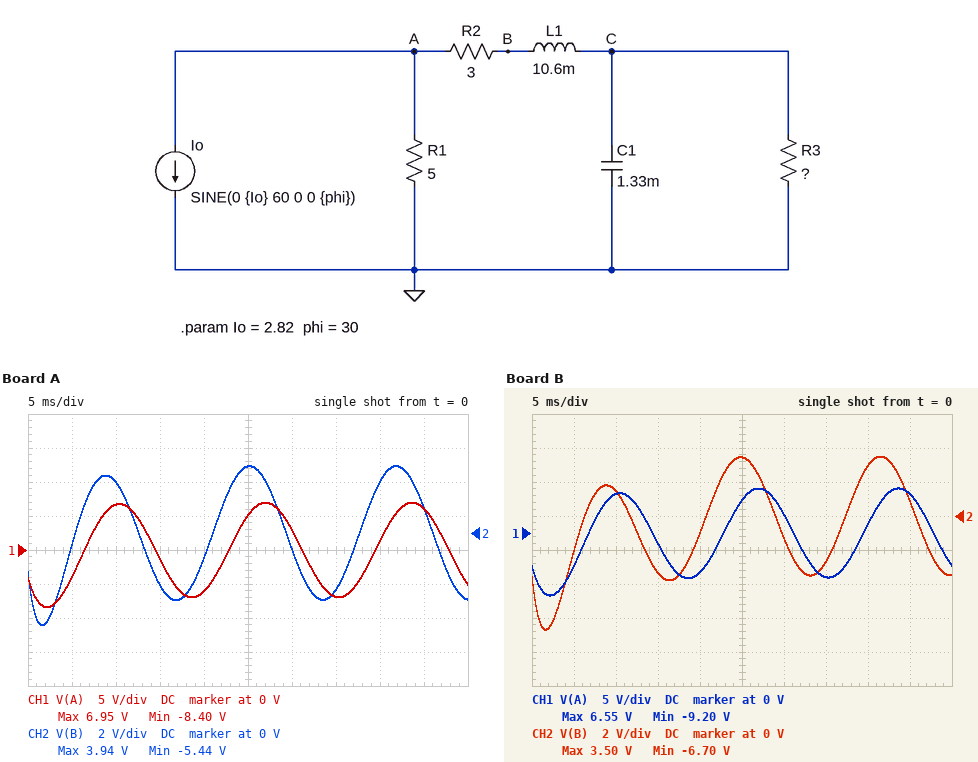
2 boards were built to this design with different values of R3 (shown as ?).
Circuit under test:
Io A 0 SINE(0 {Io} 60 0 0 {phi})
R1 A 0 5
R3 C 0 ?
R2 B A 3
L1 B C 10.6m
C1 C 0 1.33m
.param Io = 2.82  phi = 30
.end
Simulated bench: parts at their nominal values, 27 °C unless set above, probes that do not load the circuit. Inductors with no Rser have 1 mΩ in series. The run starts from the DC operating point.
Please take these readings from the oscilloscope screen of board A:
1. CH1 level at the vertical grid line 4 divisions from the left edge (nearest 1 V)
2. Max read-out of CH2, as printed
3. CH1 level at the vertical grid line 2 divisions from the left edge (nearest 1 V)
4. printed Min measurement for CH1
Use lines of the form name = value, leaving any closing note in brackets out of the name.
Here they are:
CH1 level at the vertical grid line 4 divisions from the left edge = -6 V
Max read-out of CH2, as printed = 3.94 V
CH1 level at the vertical grid line 2 divisions from the left edge = 7 V
printed Min measurement for CH1 = -8.40 V
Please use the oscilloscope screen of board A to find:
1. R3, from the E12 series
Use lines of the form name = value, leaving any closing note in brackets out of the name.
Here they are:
R3, from the E12 series = 3.9 Ω
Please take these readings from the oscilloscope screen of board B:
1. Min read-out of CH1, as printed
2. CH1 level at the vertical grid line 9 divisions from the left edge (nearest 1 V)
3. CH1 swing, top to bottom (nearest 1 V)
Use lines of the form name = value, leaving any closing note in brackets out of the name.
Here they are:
Min read-out of CH1, as printed = -9.20 V
CH1 level at the vertical grid line 9 divisions from the left edge = 6 V
CH1 swing, top to bottom = 16 V
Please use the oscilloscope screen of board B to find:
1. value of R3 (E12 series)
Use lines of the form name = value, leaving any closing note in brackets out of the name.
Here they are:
value of R3 = 8.2 Ω
